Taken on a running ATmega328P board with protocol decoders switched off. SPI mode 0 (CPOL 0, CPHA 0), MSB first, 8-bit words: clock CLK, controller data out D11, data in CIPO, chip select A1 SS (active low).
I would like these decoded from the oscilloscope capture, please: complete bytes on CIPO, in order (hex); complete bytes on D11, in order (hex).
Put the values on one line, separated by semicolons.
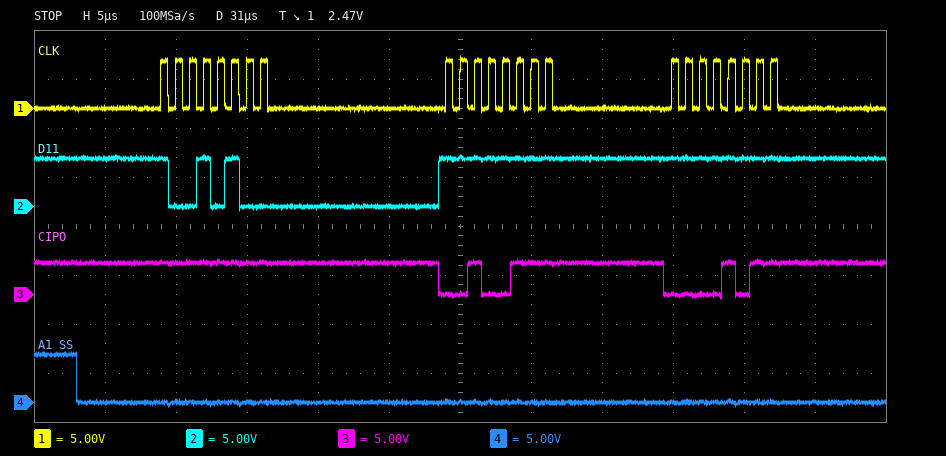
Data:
FF 27 0B; 94 FF FF
